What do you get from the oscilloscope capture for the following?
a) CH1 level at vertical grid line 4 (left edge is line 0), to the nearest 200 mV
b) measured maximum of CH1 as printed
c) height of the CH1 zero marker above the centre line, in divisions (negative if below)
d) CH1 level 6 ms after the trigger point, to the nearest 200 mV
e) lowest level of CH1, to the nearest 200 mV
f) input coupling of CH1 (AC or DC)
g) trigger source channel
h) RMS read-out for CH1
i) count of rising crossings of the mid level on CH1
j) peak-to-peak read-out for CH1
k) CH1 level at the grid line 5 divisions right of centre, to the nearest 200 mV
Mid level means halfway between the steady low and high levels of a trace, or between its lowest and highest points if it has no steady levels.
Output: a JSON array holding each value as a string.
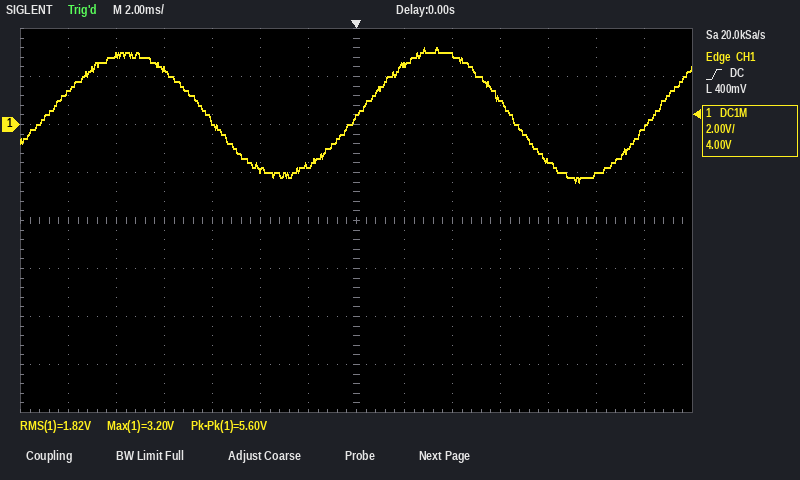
["200 mV", "3.20 V", "+2.0 div", "1.0 V", "-2.4 V", "DC", "CH1", "1.82 V", "3", "5.60 V", "-2.0 V"]
